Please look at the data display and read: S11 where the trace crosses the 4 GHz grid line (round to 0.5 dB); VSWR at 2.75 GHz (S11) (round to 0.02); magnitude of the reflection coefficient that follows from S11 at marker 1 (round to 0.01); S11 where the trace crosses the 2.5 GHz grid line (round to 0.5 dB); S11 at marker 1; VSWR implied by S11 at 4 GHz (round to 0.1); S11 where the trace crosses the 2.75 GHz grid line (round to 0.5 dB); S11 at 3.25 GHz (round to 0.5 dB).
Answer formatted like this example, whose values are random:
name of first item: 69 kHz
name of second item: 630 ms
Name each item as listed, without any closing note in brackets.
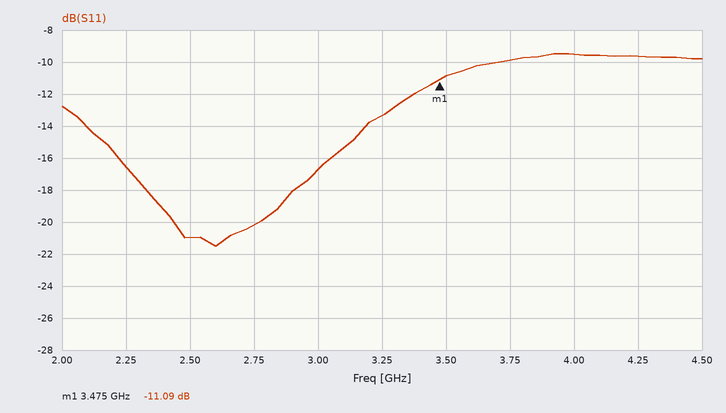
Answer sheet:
S11 where the trace crosses the 4 GHz grid line: -9.5 dB
VSWR at 2.75 GHz (S11): 1.22
magnitude of the reflection coefficient that follows from S11 at marker 1: 0.28
S11 where the trace crosses the 2.5 GHz grid line: -21.0 dB
S11 at marker 1: -11.09 dB
VSWR implied by S11 at 4 GHz: 2.0
S11 where the trace crosses the 2.75 GHz grid line: -20.0 dB
S11 at 3.25 GHz: -13.5 dB
